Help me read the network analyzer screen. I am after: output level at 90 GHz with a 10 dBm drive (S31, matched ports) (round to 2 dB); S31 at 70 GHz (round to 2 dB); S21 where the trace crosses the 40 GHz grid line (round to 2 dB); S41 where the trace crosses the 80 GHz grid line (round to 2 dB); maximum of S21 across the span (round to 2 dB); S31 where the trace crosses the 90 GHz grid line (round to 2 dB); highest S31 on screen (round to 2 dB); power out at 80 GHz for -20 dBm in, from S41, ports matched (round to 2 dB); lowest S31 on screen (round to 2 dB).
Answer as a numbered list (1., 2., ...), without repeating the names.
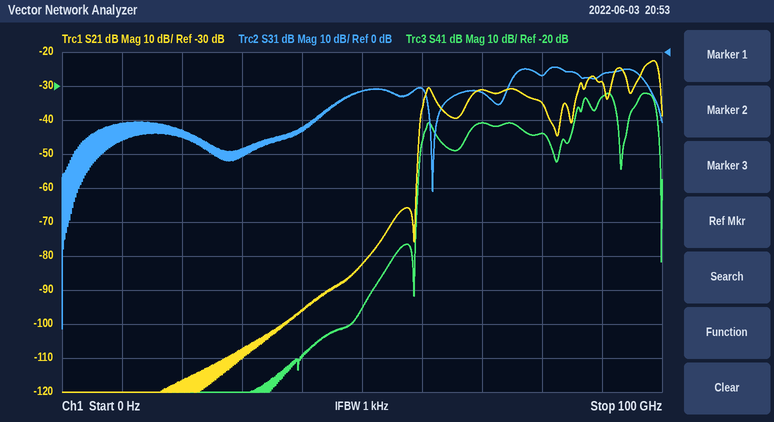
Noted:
1. 4 dBm
2. -12 dB
3. -96 dB
4. -34 dB
5. -22 dB
6. -6 dB
7. -4 dB
8. -54 dBm
9. -82 dB
